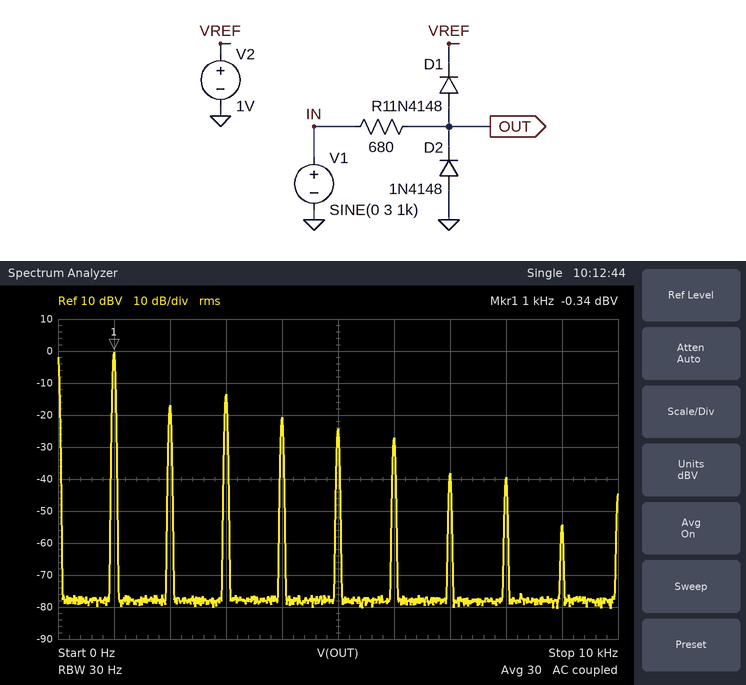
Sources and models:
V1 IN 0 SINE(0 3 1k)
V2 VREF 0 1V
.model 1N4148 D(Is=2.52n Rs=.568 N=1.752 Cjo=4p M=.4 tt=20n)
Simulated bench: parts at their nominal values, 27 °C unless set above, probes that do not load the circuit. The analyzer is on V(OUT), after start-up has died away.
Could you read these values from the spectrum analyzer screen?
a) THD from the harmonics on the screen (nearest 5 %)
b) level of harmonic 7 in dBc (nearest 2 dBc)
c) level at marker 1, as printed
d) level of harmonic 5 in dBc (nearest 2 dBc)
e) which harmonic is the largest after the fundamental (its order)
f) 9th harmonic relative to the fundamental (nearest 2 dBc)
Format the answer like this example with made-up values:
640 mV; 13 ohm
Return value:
30 %; -38 dBc; -0.34 dBV; -24 dBc; 3; -54 dBc
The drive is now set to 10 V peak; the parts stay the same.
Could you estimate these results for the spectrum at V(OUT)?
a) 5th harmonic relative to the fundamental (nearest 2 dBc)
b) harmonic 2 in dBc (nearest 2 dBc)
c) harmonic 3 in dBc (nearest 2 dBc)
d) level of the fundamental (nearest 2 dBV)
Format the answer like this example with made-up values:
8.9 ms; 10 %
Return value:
-16 dBc; -26 dBc; -10 dBc; 0 dBV
